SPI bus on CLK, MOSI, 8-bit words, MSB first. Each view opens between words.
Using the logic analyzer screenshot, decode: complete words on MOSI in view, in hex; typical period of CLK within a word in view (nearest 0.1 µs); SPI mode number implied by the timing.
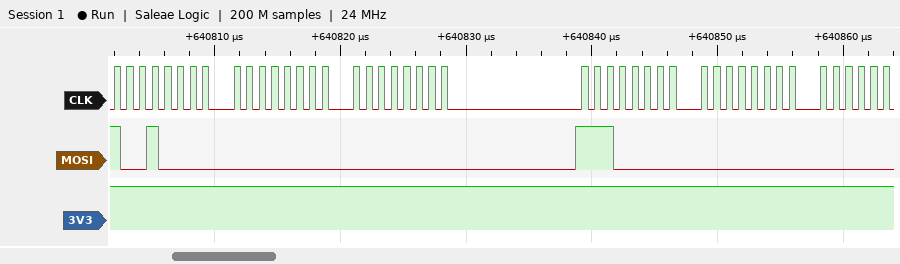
90, 00, 00, E0, 00
1 µs
0
